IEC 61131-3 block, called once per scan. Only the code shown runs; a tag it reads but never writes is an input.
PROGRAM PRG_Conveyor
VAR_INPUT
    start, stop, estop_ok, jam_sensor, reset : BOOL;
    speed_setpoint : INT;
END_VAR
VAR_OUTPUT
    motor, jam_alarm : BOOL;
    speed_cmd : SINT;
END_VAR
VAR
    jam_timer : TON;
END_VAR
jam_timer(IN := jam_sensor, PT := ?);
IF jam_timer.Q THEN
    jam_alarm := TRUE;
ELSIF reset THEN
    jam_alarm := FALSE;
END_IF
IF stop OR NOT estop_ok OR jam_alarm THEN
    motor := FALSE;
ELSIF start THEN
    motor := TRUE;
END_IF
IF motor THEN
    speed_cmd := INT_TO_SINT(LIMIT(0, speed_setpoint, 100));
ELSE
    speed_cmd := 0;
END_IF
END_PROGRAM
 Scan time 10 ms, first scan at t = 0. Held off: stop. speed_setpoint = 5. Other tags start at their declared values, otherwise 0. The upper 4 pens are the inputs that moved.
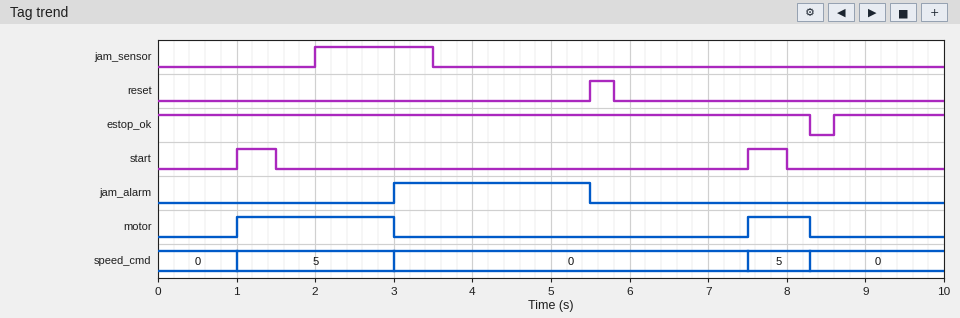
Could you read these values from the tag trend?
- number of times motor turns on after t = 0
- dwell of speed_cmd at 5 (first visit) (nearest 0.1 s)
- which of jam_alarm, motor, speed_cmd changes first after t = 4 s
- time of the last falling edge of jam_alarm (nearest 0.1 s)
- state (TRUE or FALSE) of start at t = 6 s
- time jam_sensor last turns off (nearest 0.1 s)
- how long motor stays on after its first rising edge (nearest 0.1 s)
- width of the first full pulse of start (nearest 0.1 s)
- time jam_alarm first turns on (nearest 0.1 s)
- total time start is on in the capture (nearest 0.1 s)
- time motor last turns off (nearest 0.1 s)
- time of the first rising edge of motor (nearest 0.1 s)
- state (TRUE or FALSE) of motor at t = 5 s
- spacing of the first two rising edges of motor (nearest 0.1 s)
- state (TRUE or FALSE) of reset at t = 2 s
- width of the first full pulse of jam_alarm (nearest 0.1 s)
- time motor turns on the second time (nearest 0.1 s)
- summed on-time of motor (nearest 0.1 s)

2
2.0 s
jam_alarm
5.5 s
FALSE
3.5 s
2.0 s
0.5 s
3.0 s
1.0 s
8.3 s
1.0 s
FALSE
6.5 s
FALSE
2.5 s
7.5 s
2.8 s
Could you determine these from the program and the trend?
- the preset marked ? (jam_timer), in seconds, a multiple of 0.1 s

1.0 s
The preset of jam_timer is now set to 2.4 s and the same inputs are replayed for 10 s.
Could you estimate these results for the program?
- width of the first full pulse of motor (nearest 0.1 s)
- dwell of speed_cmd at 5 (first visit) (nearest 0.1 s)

7.3 s
7.3 s
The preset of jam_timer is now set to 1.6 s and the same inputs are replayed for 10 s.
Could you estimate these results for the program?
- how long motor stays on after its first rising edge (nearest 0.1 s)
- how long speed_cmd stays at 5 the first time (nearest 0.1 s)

7.3 s
7.3 s
